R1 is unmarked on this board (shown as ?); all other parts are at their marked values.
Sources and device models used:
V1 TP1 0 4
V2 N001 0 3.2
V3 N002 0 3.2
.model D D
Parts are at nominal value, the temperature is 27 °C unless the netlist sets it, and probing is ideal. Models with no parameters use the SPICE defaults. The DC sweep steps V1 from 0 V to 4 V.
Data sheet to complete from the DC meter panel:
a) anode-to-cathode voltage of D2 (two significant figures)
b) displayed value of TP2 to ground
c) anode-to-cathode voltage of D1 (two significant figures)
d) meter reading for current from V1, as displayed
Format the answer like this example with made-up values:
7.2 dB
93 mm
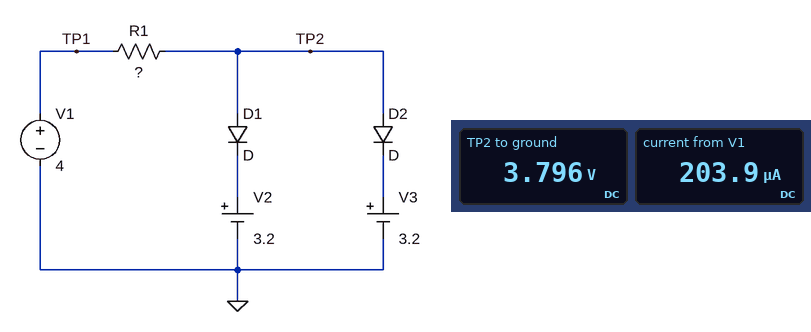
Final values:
600 mV
3.796 V
600 mV
203.9 µA
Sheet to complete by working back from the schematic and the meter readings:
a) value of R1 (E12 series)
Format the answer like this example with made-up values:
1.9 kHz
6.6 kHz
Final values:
1 kΩ
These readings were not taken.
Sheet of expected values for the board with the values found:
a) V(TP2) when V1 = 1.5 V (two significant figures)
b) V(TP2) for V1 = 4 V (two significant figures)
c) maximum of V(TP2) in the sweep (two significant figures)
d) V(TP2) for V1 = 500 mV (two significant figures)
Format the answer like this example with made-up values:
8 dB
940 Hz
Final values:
1.5 V
3.8 V
3.8 V
500 mV
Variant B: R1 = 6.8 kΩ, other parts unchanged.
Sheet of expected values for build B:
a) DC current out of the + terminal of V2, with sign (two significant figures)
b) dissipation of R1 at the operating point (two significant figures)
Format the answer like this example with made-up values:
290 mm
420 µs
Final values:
-18 µA
9.1 µW
